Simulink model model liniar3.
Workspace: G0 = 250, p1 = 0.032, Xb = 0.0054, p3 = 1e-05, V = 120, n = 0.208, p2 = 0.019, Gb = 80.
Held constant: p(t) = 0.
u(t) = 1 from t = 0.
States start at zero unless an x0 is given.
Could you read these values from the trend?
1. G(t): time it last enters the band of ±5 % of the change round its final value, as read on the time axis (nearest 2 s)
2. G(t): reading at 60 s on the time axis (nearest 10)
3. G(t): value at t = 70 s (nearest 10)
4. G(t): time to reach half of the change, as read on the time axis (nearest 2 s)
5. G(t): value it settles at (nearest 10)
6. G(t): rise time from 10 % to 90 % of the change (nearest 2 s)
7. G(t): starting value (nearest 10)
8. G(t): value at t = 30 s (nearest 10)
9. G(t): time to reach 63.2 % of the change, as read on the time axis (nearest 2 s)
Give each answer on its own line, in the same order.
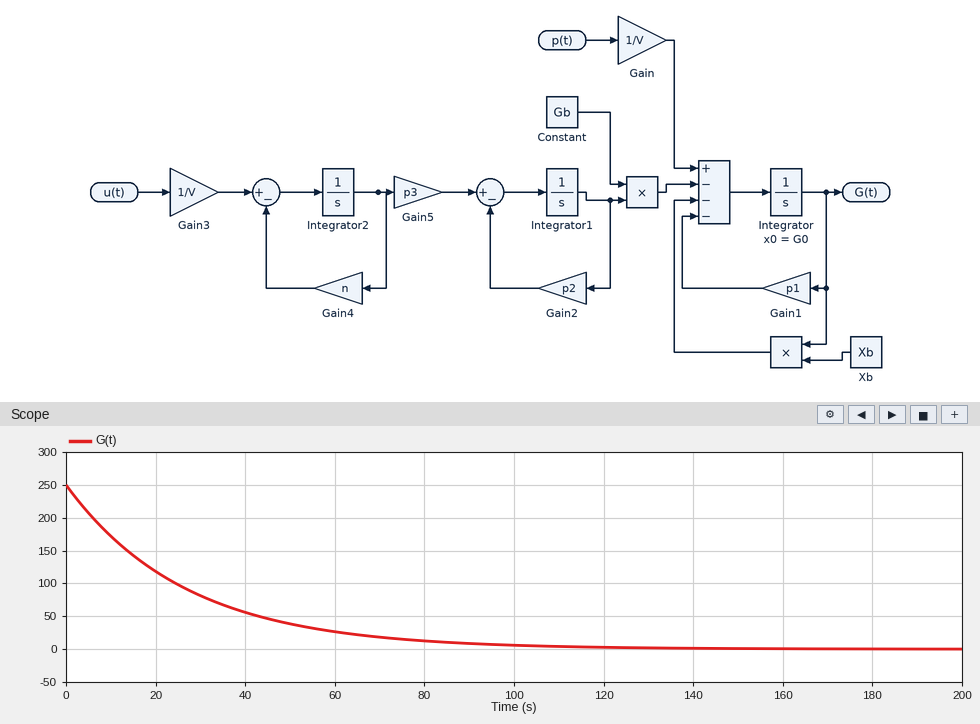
80 s
30
20
18 s
0
58 s
250
80
26 s
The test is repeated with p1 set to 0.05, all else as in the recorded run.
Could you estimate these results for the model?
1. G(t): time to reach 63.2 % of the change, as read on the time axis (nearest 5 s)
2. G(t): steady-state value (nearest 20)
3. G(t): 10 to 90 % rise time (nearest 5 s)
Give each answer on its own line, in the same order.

20 s
0
40 s
